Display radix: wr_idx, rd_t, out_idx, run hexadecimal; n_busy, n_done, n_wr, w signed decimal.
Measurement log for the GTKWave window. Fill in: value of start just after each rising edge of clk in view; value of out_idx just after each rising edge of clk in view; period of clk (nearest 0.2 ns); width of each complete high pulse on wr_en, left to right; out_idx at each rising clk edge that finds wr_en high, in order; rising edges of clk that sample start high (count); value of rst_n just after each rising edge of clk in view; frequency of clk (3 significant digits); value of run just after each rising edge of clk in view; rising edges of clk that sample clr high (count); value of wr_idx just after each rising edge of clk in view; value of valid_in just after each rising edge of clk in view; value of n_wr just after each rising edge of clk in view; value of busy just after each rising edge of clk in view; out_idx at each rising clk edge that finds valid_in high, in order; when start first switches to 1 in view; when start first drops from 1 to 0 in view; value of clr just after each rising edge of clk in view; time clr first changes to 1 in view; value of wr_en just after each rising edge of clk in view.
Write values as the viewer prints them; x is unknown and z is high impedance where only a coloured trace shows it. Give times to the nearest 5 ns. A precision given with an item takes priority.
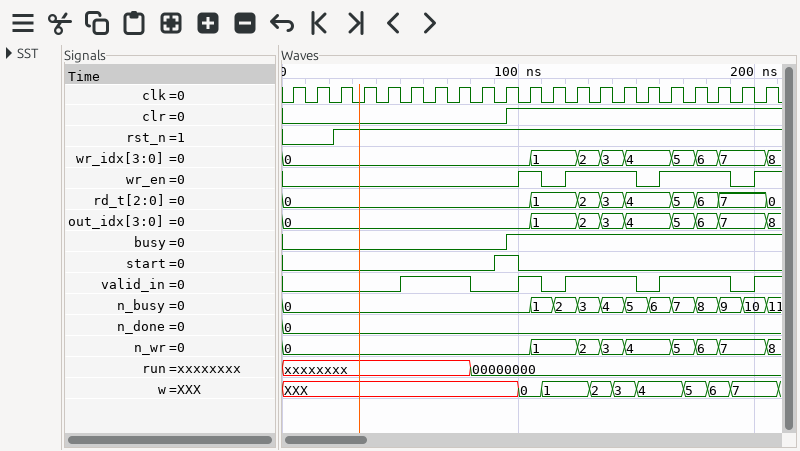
0 0 0 0 0 0 0 0 0 1 0 0 0 0 0 0 0 0 0 0 0
0, 0, 0, 0, 0, 0, 0, 0, 0, 0, 1, 1, 2, 3, 4, 4, 5, 6, 7, 7, 8
10 ns
10 ns, 30 ns, 30 ns
0, 1, 2, 3, 4, 5, 6, 7
1
0 0 1 1 1 1 1 1 1 1 1 1 1 1 1 1 1 1 1 1 1
100 MHz
xxxxxxxx, xxxxxxxx, xxxxxxxx, xxxxxxxx, xxxxxxxx, xxxxxxxx, xxxxxxxx, xxxxxxxx, 00000000, 00000000, 00000000, 00000000, 00000000, 00000000, 00000000, 00000000, 00000000, 00000000, 00000000, 00000000, 00000000
11
0, 0, 0, 0, 0, 0, 0, 0, 0, 0, 1, 1, 2, 3, 4, 4, 5, 6, 7, 7, 8
0 0 0 0 0 1 1 1 0 0 1 0 1 1 1 0 1 1 1 0 1
0, 0, 0, 0, 0, 0, 0, 0, 0, 0, 1, 1, 2, 3, 4, 4, 5, 6, 7, 7, 8
0 0 0 0 0 0 0 0 0 1 1 1 1 1 1 1 1 1 1 1 1
0, 0, 0, 0, 1, 2, 3, 4, 5, 6, 7
90 ns
100 ns
0 0 0 0 0 0 0 0 0 1 1 1 1 1 1 1 1 1 1 1 1
95 ns
0 0 0 0 0 0 0 0 0 0 1 0 1 1 1 0 1 1 1 0 1
